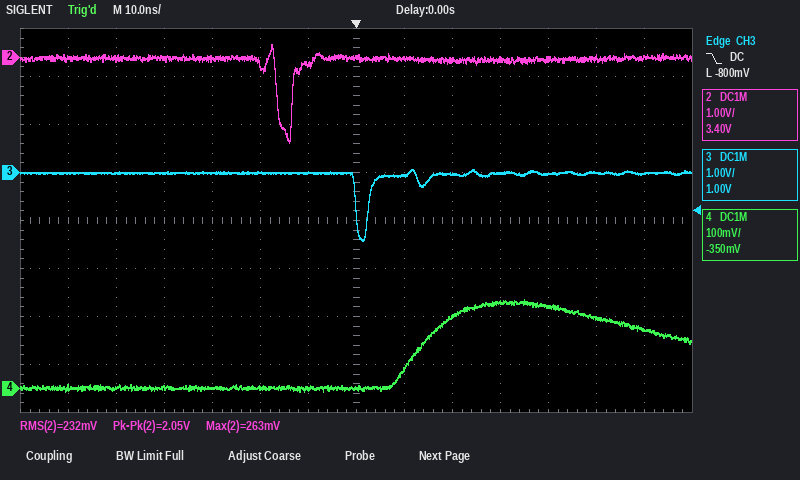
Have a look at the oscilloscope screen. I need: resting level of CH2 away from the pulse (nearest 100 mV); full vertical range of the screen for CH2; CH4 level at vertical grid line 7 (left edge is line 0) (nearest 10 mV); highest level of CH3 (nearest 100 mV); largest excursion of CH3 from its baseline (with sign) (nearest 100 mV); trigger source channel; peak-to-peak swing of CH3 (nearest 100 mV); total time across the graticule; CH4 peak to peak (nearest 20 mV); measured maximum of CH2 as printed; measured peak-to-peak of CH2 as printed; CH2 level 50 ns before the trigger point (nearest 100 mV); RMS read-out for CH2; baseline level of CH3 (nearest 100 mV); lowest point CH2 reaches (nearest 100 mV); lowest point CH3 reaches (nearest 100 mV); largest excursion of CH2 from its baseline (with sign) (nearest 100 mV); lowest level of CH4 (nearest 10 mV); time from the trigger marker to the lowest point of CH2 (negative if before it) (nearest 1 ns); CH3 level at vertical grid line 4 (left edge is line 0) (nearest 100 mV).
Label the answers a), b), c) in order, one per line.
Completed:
a) 0.0 V
b) 8 V
c) 0 mV
d) 100 mV
e) -1.4 V
f) CH3
g) 1.5 V
h) 140 ns
i) 200 mV
j) 263 mV
k) 2.05 V
l) 0.0 V
m) 232 mV
n) 0.0 V
o) -1.8 V
p) -1.4 V
q) -1.8 V
r) -10 mV
s) -14 ns
t) 0.0 V
